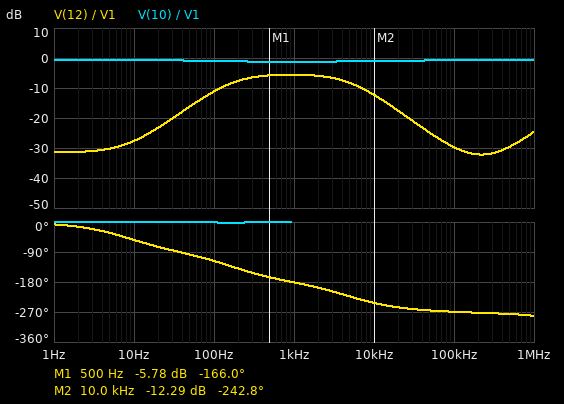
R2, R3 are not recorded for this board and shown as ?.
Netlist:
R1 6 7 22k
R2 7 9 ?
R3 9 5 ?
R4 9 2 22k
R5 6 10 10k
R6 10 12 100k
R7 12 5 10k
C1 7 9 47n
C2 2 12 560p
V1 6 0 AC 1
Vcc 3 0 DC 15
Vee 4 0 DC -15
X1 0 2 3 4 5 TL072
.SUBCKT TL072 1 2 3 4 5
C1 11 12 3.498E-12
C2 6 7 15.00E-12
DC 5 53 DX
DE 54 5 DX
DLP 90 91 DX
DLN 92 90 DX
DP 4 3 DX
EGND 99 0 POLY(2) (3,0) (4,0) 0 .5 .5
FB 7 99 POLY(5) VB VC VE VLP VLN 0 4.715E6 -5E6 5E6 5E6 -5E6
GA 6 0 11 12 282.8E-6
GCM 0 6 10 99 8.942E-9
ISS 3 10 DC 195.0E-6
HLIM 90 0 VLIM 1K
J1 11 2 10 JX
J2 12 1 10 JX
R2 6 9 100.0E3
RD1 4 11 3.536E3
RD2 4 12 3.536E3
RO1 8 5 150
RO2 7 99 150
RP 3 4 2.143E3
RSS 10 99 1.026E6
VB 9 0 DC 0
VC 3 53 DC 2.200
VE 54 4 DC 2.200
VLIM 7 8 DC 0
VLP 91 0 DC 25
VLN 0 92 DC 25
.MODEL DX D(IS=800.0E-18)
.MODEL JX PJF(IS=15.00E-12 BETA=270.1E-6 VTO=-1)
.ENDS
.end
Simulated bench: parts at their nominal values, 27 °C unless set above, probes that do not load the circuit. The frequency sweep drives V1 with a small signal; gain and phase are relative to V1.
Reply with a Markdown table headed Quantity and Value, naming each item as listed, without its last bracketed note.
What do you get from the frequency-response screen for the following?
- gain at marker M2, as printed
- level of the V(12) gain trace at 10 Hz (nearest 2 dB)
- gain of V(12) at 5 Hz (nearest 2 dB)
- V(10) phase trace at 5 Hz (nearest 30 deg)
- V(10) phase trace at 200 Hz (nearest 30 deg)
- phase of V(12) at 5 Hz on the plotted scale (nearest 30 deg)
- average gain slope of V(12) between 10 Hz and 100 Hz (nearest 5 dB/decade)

| Quantity | Value |
|---|---|
| gain at marker M2, as printed | -12.29 dB |
| level of the V(12) gain trace at 10 Hz | -28 dB |
| gain of V(12) at 5 Hz | -30 dB |
| V(10) phase trace at 5 Hz | 0 deg |
| V(10) phase trace at 200 Hz | 0 deg |
| phase of V(12) at 5 Hz on the plotted scale | -30 deg |
| average gain slope of V(12) between 10 Hz and 100 Hz | 15 dB/decade |
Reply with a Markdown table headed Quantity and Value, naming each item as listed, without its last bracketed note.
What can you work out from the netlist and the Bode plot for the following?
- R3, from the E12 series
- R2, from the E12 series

| Quantity | Value |
|---|---|
| R3, from the E12 series | 15 kΩ |
| R2, from the E12 series | 220 kΩ |
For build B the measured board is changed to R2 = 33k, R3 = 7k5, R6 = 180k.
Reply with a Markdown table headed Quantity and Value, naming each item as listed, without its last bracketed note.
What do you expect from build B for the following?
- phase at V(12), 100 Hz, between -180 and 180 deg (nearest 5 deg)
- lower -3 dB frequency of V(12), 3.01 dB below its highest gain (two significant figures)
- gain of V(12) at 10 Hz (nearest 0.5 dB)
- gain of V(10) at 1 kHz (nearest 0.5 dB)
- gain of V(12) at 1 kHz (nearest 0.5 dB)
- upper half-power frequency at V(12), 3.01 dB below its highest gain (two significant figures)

| Quantity | Value |
|---|---|
| phase at V(12), 100 Hz, between -180 and 180 deg | -150 deg |
| lower -3 dB frequency of V(12), 3.01 dB below its highest gain | 220 Hz |
| gain of V(12) at 10 Hz | -22.0 dB |
| gain of V(10) at 1 kHz | -0.5 dB |
| gain of V(12) at 1 kHz | -11.5 dB |
| upper half-power frequency at V(12), 3.01 dB below its highest gain | 6.8 kHz |
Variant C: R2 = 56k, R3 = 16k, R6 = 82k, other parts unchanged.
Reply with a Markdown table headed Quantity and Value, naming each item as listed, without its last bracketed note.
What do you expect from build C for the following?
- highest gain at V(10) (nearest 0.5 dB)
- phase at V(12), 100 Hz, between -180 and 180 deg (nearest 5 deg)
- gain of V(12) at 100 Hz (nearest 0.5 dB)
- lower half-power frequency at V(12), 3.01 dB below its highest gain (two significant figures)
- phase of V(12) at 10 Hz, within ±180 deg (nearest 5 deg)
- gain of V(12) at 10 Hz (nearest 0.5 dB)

| Quantity | Value |
|---|---|
| highest gain at V(10) | -1.0 dB |
| phase at V(12), 100 Hz, between -180 and 180 deg | -135 deg |
| gain of V(12) at 100 Hz | -12.0 dB |
| lower half-power frequency at V(12), 3.01 dB below its highest gain | 190 Hz |
| phase of V(12) at 10 Hz, within ±180 deg | -165 deg |
| gain of V(12) at 10 Hz | -21.0 dB |
